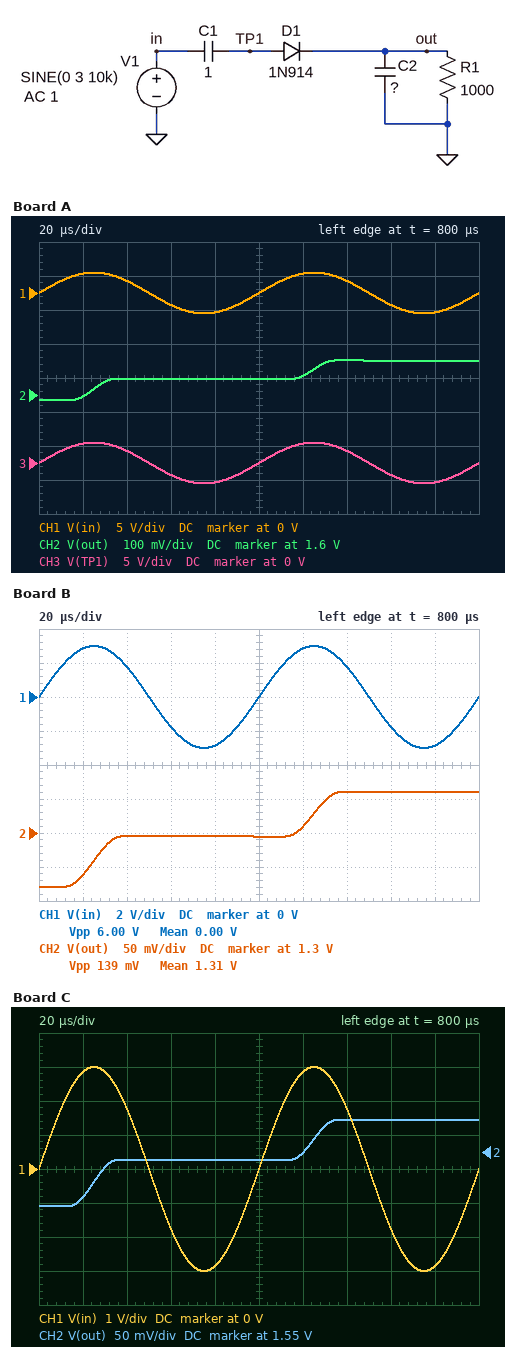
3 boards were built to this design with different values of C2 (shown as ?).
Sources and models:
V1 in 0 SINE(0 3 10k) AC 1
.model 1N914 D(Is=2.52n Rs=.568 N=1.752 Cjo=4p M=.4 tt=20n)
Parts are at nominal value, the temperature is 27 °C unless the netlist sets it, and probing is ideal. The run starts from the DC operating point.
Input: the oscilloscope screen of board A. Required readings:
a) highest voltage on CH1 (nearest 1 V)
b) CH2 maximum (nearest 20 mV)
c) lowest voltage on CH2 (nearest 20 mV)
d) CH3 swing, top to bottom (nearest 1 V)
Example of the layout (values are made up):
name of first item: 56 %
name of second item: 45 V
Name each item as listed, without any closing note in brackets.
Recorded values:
highest voltage on CH1: 3 V
CH2 maximum: 1.70 V
lowest voltage on CH2: 1.58 V
CH3 swing, top to bottom: 6 V
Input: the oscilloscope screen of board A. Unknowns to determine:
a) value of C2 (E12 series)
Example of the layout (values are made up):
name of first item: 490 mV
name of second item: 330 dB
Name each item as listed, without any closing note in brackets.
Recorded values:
value of C2: 180 µF
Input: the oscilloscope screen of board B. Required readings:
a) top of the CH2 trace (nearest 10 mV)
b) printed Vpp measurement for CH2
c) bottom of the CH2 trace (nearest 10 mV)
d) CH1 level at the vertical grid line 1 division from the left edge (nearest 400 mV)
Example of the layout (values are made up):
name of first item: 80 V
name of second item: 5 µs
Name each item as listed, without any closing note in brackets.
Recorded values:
top of the CH2 trace: 1.36 V
printed Vpp measurement for CH2: 139 mV
bottom of the CH2 trace: 1.22 V
CH1 level at the vertical grid line 1 division from the left edge: 2.8 V
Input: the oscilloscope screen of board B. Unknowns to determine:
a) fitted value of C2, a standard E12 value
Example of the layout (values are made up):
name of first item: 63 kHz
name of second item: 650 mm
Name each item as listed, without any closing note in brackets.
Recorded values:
fitted value of C2, a standard E12 value: 330 µF
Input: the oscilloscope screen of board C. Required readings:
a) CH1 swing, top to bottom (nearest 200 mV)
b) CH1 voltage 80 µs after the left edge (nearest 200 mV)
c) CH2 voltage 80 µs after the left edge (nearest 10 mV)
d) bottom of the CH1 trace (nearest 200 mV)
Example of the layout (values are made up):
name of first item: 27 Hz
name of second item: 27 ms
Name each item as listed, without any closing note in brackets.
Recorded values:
CH1 swing, top to bottom: 6.0 V
CH1 voltage 80 µs after the left edge: -2.8 V
CH2 voltage 80 µs after the left edge: 1.54 V
bottom of the CH1 trace: -3.0 V
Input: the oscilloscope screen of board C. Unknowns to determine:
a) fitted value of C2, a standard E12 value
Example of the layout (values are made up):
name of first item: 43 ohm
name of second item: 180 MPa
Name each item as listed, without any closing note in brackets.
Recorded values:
fitted value of C2, a standard E12 value: 220 µF
